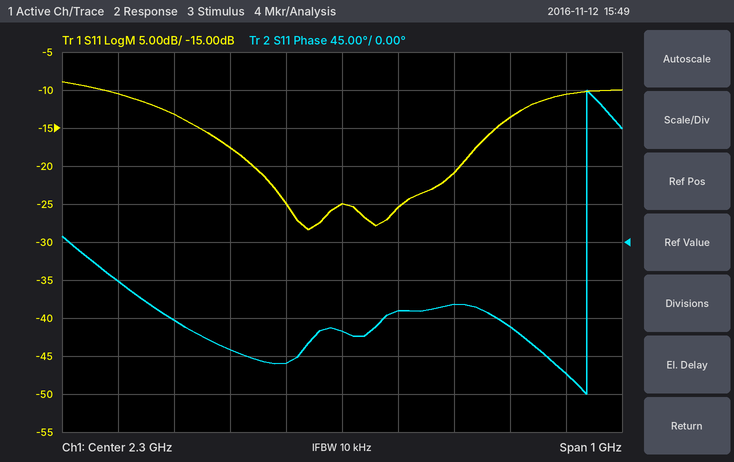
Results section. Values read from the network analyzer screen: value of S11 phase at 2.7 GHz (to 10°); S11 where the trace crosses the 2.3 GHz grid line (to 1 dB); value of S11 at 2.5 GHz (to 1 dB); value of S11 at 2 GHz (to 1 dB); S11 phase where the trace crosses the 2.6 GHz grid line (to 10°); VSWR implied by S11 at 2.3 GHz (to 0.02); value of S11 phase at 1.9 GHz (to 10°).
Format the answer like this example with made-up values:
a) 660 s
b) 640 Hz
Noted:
a) -160°
b) -25 dB
c) -21 dB
d) -13 dB
e) -100°
f) 1.12
g) -50°
